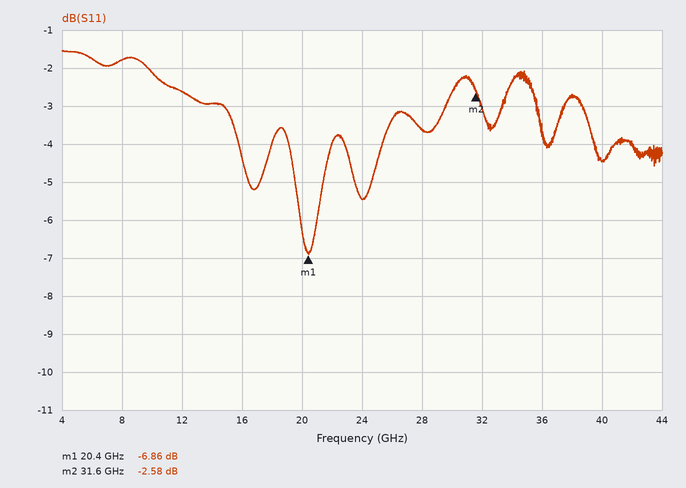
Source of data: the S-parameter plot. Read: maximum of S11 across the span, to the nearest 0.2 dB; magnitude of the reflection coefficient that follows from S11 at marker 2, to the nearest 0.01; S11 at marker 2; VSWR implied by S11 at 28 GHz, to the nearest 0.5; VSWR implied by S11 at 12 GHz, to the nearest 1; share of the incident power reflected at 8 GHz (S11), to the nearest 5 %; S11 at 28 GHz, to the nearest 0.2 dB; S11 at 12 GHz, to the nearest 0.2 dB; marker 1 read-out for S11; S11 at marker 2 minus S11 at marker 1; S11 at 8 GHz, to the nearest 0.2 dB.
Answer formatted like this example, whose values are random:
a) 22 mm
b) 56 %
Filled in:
a) -1.6 dB
b) 0.74
c) -2.58 dB
d) 5.0
e) 7
f) 65 %
g) -3.6 dB
h) -2.6 dB
i) -6.86 dB
j) 4.28 dB
k) -1.8 dB
